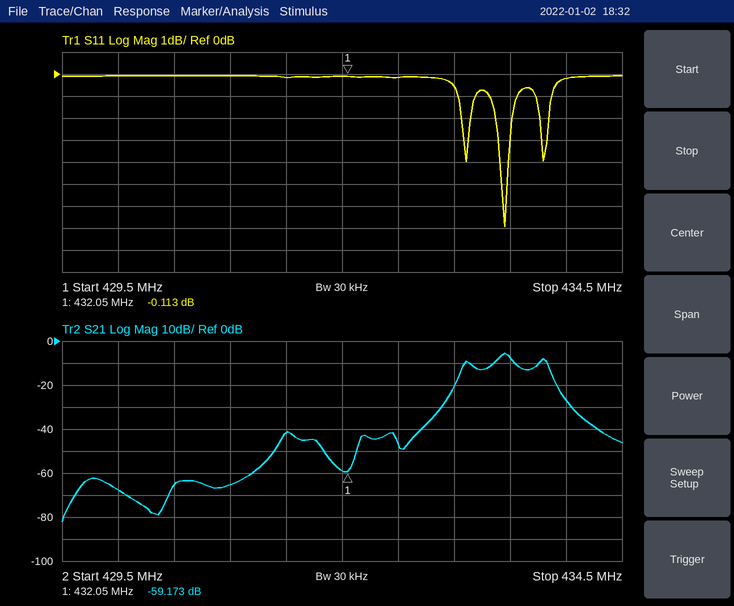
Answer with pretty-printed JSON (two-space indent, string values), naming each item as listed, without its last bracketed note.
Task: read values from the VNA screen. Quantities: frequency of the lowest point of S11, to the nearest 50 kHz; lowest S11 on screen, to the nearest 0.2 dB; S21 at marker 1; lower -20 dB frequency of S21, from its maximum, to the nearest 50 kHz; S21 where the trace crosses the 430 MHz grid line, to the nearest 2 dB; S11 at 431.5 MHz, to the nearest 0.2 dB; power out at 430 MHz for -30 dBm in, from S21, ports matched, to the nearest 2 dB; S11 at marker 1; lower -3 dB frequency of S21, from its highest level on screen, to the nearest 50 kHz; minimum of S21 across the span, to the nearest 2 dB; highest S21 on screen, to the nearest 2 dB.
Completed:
{
  "frequency of the lowest point of S11, to the nearest 50 kHz": "433.45 MHz",
  "lowest S11 on screen, to the nearest 0.2 dB": "-7.0 dB",
  "S21 at marker 1": "-59.173 dB",
  "lower -20 dB frequency of S21, from its maximum, to the nearest 50 kHz": "432.95 MHz",
  "S21 where the trace crosses the 430 MHz grid line, to the nearest 2 dB": "-68 dB",
  "S11 at 431.5 MHz, to the nearest 0.2 dB": "-0.2 dB",
  "power out at 430 MHz for -30 dBm in, from S21, ports matched, to the nearest 2 dB": "-98 dBm",
  "S11 at marker 1": "-0.113 dB",
  "lower -3 dB frequency of S21, from its highest level on screen, to the nearest 50 kHz": "433.40 MHz",
  "minimum of S21 across the span, to the nearest 2 dB": "-82 dB",
  "highest S21 on screen, to the nearest 2 dB": "-6 dB"
}
